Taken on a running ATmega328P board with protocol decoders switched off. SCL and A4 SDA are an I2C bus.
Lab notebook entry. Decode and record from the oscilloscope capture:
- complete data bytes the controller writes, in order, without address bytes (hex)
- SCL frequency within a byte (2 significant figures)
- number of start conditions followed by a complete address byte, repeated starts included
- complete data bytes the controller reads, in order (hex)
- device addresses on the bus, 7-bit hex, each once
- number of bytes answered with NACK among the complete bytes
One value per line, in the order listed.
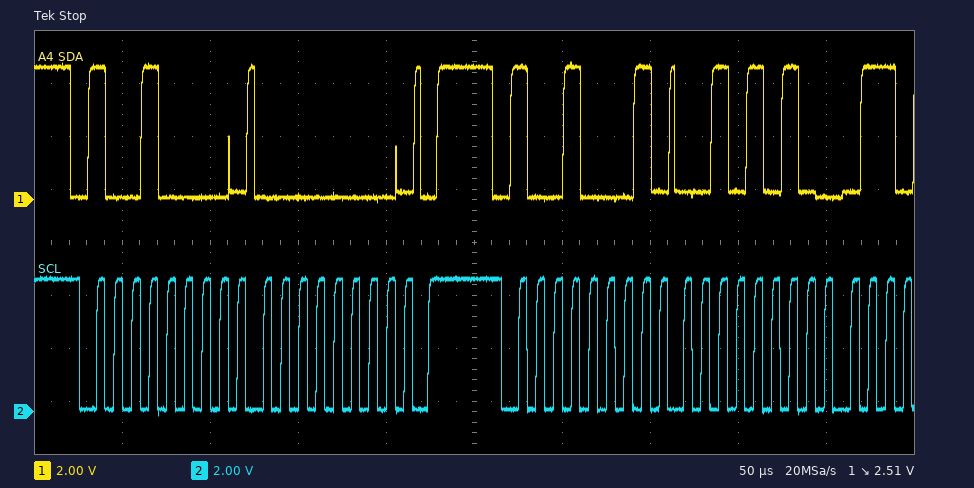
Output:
00
100 kHz
2
2A
0x48
0
